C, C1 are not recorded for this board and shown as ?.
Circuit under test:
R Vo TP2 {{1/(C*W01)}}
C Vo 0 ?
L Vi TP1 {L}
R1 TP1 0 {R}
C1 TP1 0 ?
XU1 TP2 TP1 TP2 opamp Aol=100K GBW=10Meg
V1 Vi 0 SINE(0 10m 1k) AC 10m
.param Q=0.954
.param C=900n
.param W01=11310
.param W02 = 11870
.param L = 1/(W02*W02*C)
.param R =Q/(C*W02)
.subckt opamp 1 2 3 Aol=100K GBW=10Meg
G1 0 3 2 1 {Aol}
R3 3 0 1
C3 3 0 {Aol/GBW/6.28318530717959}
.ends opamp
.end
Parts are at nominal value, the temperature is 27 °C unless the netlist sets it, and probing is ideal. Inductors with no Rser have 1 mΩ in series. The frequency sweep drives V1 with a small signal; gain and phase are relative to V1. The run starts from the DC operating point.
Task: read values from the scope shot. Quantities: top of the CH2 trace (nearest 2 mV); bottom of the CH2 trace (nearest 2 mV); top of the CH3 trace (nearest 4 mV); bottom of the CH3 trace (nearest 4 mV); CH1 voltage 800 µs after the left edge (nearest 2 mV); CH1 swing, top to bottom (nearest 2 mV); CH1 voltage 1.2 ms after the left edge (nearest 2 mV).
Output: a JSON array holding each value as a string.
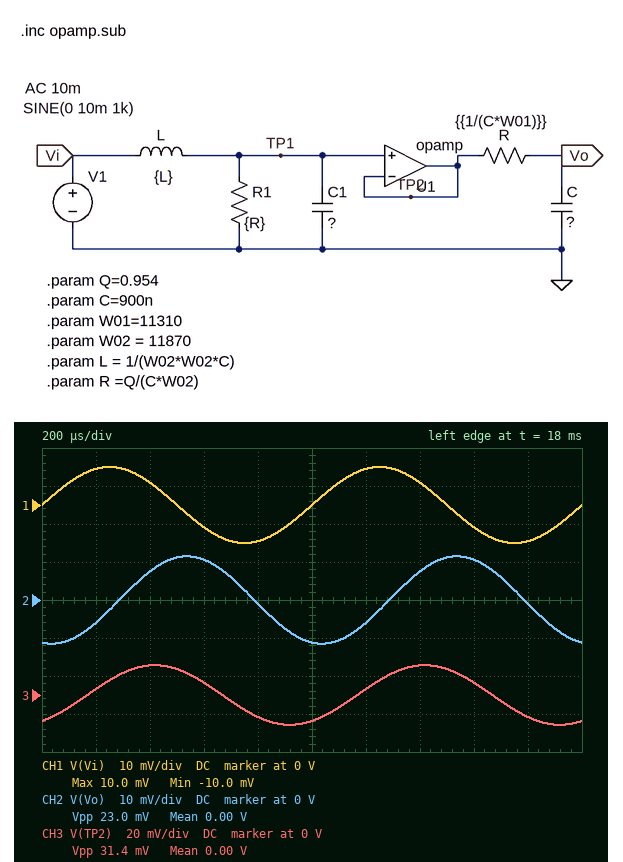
["12 mV", "-12 mV", "16 mV", "-16 mV", "-10 mV", "20 mV", "10 mV"]
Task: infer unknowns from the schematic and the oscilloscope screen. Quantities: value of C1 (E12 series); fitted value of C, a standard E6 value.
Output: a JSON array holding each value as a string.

["2.2 µF", "1.5 µF"]
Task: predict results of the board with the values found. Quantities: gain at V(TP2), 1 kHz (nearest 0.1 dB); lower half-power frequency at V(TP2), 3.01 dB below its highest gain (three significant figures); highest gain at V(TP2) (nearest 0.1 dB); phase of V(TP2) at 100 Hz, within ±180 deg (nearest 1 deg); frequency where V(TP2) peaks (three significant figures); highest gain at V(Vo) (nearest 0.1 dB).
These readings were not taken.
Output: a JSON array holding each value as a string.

["3.9 dB", "458 Hz", "4.0 dB", "-3 deg", "1.06 kHz", "1.2 dB"]
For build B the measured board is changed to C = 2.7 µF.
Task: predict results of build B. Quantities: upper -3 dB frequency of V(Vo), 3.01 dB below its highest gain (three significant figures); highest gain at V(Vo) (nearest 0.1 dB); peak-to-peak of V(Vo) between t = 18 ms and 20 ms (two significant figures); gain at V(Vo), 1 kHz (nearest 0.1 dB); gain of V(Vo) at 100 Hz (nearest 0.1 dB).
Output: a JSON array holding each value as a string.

["1.16 kHz", "0 dB", "16 mV", "-1.9 dB", "-0.1 dB"]
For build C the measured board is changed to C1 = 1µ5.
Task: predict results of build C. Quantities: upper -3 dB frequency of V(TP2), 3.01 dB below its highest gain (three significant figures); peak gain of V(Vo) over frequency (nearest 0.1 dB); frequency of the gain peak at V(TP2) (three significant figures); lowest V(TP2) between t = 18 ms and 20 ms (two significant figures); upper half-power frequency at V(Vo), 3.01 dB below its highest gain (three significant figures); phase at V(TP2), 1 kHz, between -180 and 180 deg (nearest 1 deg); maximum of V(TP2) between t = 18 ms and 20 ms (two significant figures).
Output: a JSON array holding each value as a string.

["1.74 kHz", "0 dB", "1.20 kHz", "-13 mV", "1.49 kHz", "-46 deg", "13 mV"]
